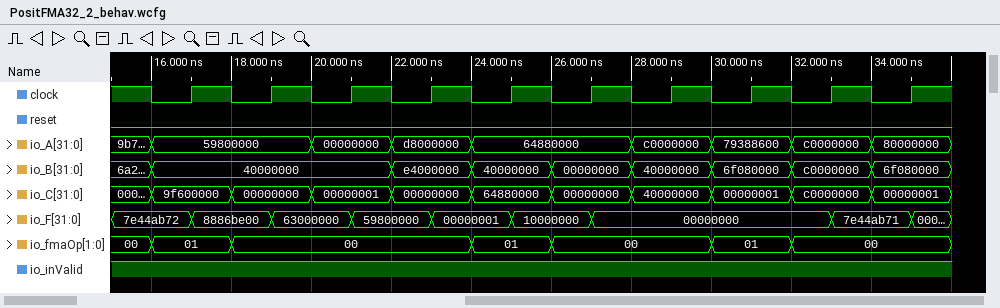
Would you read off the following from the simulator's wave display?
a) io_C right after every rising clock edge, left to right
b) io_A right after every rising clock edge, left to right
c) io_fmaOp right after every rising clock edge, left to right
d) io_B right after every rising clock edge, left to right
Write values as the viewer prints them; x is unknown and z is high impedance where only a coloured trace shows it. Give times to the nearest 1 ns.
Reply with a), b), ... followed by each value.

a) 9f600000, 00000000, 00000001, 00000000, 64880000, 00000000, 40000000, 00000001, c0000000, 00000001
b) 59800000, 59800000, 00000000, d8000000, 64880000, 64880000, c0000000, 79388600, c0000000, 80000000
c) 01, 00, 00, 00, 01, 00, 00, 01, 00, 00
d) 40000000, 40000000, 40000000, e4000000, 40000000, 00000000, 40000000, 6f080000, c0000000, 6f080000
